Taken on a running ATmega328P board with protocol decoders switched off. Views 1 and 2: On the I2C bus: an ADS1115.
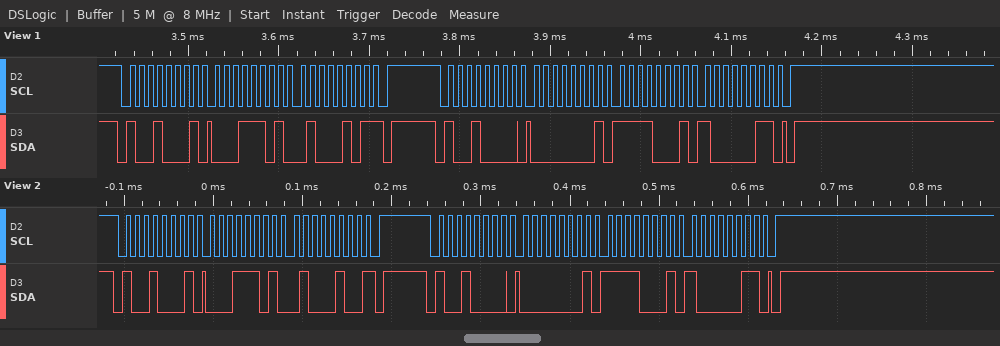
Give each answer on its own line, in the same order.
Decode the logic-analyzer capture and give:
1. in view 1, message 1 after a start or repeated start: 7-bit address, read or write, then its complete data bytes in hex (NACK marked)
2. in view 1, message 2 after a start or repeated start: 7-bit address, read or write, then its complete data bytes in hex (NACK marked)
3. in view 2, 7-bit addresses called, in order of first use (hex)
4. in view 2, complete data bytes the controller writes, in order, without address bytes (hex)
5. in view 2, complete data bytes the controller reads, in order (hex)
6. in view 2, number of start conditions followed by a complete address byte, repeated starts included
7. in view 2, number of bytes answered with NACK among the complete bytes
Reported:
0x48 read: 1D 45 NACK
0x48 write: 01 F1 83
0x48
01 F1 83
1D 44
2
1
